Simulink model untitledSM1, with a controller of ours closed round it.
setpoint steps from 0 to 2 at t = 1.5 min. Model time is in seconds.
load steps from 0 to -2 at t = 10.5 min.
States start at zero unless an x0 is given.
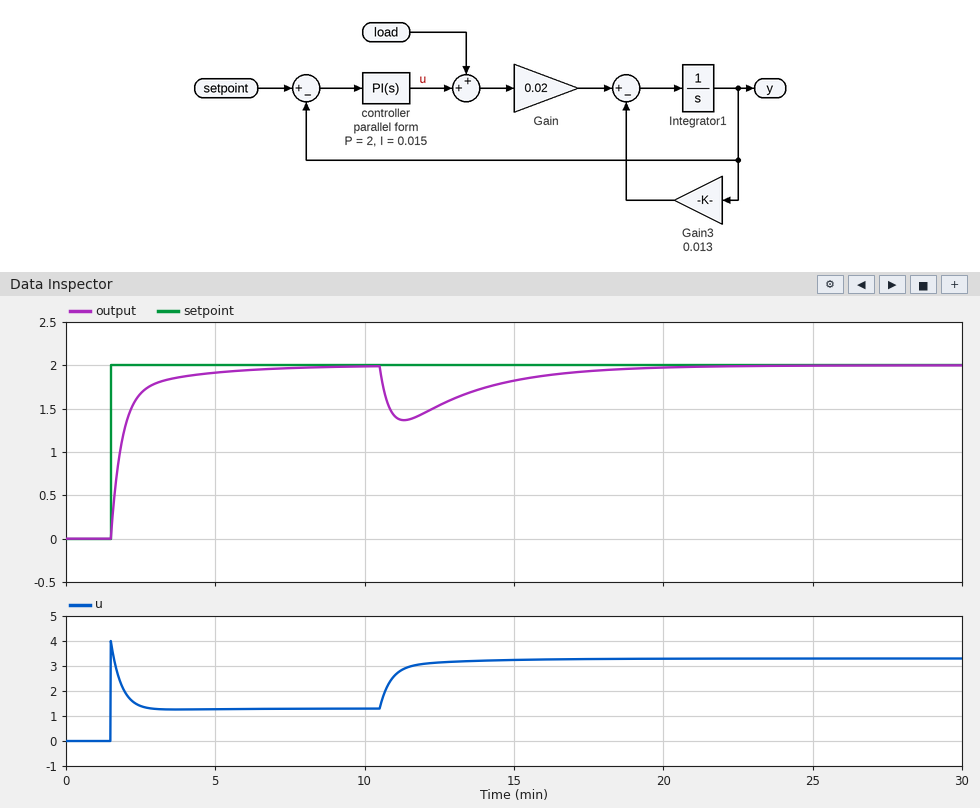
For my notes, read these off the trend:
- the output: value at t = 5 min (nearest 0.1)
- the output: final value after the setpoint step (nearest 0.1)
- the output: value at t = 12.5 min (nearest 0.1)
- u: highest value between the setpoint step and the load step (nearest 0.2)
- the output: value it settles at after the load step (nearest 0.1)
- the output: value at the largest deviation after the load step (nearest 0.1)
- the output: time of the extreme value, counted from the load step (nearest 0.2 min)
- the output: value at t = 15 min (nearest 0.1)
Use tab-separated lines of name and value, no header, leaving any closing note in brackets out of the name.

the output: value at t = 5 min	1.9
the output: final value after the setpoint step	2.0
the output: value at t = 12.5 min	1.5
u: highest value between the setpoint step and the load step	4.0
the output: value it settles at after the load step	2.0
the output: value at the largest deviation after the load step	1.4
the output: time of the extreme value, counted from the load step	0.8 min
the output: value at t = 15 min	1.8
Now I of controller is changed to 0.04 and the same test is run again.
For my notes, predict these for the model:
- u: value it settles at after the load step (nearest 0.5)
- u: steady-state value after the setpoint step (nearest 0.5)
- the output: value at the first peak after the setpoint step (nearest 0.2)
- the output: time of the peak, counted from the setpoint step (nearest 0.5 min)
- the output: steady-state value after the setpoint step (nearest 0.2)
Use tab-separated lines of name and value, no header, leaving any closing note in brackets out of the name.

u: value it settles at after the load step	3.5
u: steady-state value after the setpoint step	1.5
the output: value at the first peak after the setpoint step	2.0
the output: time of the peak, counted from the setpoint step	1.5 min
the output: steady-state value after the setpoint step	2.0
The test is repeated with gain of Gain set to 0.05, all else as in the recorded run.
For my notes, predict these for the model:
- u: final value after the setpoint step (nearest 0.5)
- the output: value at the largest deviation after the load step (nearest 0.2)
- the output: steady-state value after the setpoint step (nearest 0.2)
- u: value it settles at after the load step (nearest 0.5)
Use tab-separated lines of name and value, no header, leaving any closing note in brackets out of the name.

u: final value after the setpoint step	0.5
the output: value at the largest deviation after the load step	1.2
the output: steady-state value after the setpoint step	2.0
u: value it settles at after the load step	2.5
